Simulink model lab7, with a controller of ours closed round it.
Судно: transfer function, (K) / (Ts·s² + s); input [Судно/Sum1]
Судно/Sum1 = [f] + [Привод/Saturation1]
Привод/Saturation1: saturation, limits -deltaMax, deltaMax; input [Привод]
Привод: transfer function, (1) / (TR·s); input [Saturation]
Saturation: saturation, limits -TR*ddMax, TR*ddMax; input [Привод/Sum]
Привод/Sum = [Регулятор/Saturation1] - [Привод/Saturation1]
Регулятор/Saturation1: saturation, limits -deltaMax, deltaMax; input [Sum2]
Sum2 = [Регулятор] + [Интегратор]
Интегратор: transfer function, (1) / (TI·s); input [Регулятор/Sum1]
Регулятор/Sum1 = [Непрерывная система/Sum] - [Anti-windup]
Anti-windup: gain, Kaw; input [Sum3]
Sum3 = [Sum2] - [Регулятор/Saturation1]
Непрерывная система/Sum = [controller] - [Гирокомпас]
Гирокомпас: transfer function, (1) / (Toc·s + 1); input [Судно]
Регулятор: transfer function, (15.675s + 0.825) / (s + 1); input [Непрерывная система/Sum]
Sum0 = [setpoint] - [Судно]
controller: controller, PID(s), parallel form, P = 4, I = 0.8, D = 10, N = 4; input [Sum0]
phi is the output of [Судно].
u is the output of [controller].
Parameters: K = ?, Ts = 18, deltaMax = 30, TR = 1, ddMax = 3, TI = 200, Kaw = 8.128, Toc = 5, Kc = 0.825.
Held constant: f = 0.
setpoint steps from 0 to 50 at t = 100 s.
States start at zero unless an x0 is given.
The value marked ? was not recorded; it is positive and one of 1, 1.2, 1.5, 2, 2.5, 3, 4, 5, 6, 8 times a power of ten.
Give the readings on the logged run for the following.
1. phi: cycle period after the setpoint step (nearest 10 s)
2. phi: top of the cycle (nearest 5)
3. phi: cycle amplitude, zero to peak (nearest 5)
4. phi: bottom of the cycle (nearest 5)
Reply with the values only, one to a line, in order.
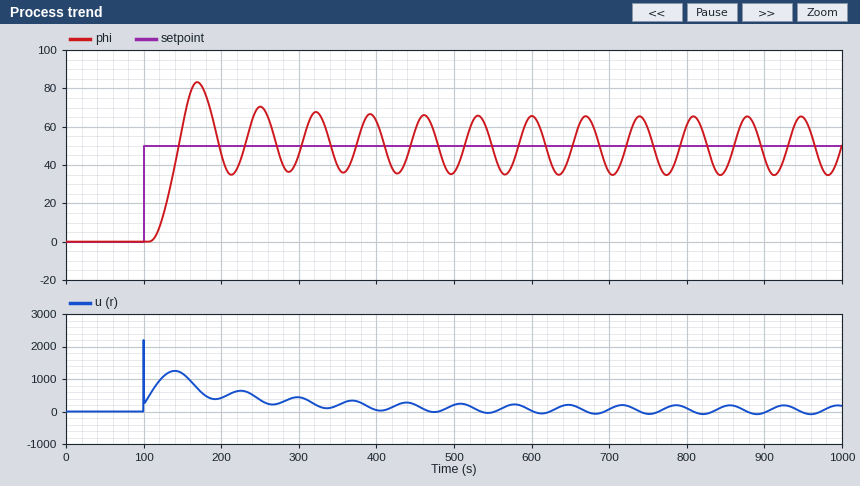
70 s
65
15
35
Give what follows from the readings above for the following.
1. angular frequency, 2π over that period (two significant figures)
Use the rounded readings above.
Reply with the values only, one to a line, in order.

0.090 rad/s
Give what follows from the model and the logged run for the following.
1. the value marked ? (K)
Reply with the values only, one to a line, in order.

0.08
